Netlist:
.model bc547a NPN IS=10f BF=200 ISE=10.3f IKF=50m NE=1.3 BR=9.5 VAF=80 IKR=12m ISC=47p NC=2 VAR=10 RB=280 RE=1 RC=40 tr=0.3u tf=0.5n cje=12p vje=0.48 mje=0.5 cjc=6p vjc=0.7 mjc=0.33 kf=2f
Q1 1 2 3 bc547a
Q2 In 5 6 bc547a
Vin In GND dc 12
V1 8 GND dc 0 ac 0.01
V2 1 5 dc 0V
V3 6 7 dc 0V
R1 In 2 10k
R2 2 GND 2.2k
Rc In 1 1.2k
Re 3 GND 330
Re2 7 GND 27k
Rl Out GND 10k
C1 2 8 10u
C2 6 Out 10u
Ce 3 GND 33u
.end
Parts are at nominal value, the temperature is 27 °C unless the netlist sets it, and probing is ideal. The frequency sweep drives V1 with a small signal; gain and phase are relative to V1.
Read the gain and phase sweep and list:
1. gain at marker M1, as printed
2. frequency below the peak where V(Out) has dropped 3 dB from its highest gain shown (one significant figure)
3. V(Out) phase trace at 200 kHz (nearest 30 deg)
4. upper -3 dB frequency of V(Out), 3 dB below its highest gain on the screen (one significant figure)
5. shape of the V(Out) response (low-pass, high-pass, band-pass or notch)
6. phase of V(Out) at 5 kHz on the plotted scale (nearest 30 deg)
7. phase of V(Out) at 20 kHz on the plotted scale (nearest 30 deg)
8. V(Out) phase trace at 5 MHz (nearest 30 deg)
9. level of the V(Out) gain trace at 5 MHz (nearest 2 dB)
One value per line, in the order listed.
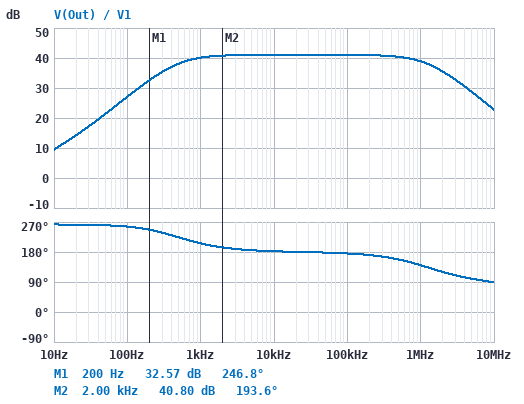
32.57 dB
500 Hz
180 deg
1 MHz
band-pass
180 deg
180 deg
90 deg
28 dB
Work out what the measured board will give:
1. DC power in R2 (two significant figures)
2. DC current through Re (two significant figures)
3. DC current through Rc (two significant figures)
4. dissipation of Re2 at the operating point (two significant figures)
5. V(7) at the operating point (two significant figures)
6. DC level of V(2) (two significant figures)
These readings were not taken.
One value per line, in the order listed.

2.0 mW
4.2 mA
4.2 mA
1.5 mW
6.3 V
2.1 V
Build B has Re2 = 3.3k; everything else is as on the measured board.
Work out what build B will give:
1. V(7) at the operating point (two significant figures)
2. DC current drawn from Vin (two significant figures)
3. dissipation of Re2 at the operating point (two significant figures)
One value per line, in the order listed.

6.3 V
7.1 mA
12 mW
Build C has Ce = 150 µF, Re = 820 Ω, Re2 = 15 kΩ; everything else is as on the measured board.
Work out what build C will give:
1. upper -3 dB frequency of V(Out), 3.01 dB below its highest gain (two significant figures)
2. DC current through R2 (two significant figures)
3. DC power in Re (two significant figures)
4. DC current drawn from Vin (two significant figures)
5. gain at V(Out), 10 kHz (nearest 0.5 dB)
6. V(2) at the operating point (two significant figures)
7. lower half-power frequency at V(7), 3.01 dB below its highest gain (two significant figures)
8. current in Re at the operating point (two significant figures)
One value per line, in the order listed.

2.2 MHz
970 µA
2.6 mW
3.4 mA
36.0 dB
2.1 V
67 Hz
1.8 mA
